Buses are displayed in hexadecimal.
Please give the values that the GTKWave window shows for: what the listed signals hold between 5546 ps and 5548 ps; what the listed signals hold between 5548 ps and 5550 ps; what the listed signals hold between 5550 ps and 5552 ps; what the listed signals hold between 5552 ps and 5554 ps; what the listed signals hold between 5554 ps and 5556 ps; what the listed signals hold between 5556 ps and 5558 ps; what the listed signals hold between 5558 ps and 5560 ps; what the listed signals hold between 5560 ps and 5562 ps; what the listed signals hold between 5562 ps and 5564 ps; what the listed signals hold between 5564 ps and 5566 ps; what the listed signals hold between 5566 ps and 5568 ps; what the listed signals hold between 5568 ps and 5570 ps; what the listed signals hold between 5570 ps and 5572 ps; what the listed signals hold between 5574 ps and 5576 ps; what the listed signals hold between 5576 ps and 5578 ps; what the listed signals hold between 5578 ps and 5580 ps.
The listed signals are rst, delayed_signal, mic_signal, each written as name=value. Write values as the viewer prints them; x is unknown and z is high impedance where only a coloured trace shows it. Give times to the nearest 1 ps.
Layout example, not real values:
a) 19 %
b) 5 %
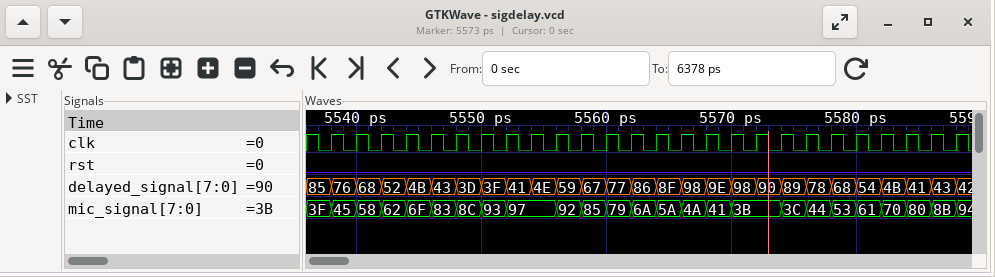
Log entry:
a) rst=0, delayed_signal=43, mic_signal=83
b) rst=0, delayed_signal=3D, mic_signal=8C
c) rst=0, delayed_signal=3F, mic_signal=93
d) rst=0, delayed_signal=41, mic_signal=97
e) rst=0, delayed_signal=4E, mic_signal=97
f) rst=0, delayed_signal=59, mic_signal=92
g) rst=0, delayed_signal=67, mic_signal=85
h) rst=0, delayed_signal=77, mic_signal=79
i) rst=0, delayed_signal=86, mic_signal=6A
j) rst=0, delayed_signal=8F, mic_signal=5A
k) rst=0, delayed_signal=98, mic_signal=4A
l) rst=0, delayed_signal=9E, mic_signal=41
m) rst=0, delayed_signal=98, mic_signal=3B
n) rst=0, delayed_signal=89, mic_signal=3C
o) rst=0, delayed_signal=78, mic_signal=44
p) rst=0, delayed_signal=68, mic_signal=53
